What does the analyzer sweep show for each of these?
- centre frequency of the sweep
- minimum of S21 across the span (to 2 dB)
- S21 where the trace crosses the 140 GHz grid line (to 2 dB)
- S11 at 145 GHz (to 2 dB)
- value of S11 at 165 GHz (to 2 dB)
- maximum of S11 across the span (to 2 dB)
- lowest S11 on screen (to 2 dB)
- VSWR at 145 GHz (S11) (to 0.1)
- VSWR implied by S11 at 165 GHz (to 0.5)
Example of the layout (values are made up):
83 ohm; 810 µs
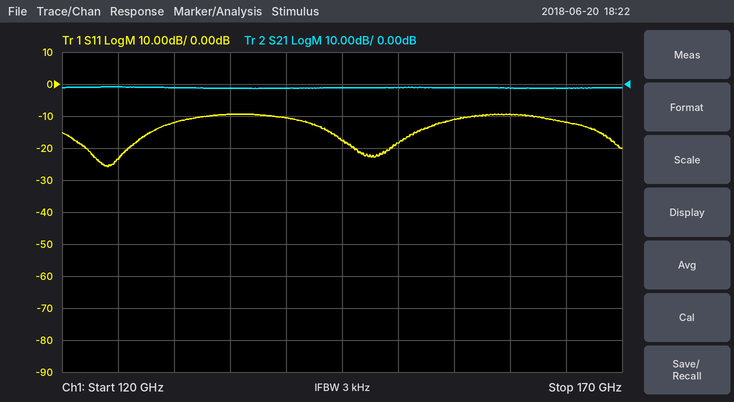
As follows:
145 GHz; -2 dB; -2 dB; -18 dB; -12 dB; -10 dB; -26 dB; 1.3; 1.5
